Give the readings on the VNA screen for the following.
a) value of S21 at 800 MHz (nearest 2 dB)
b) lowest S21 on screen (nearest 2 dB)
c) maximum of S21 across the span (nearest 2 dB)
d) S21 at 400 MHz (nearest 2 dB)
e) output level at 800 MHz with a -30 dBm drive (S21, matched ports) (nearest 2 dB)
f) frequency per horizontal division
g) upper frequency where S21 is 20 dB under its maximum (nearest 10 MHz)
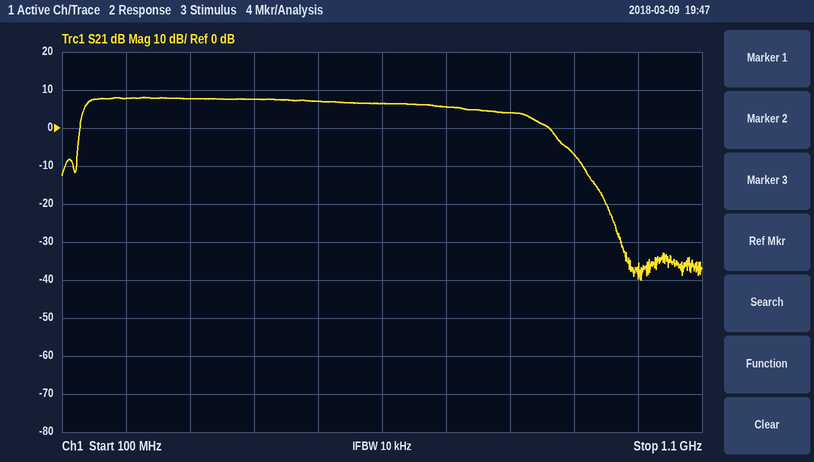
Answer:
4 dB
-40 dB
8 dB
8 dB
-26 dBm
100 MHz
920 MHz
